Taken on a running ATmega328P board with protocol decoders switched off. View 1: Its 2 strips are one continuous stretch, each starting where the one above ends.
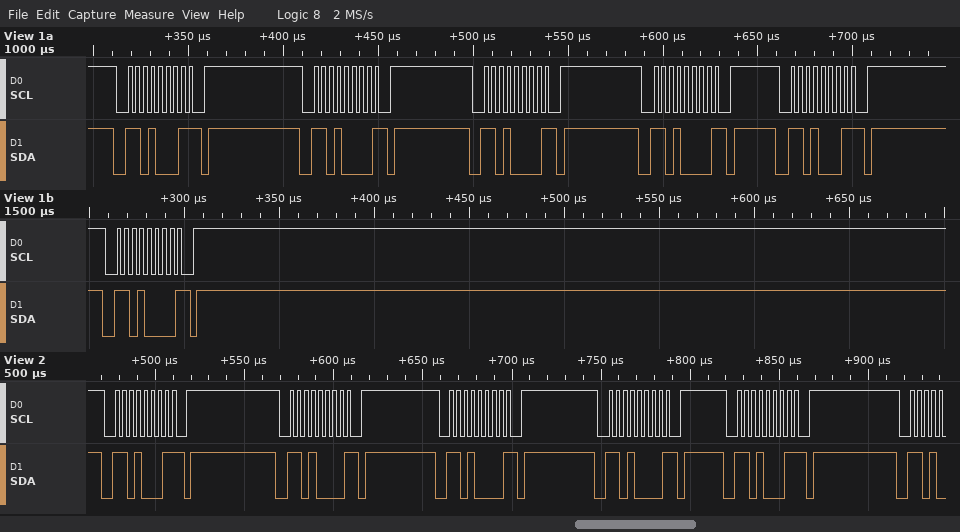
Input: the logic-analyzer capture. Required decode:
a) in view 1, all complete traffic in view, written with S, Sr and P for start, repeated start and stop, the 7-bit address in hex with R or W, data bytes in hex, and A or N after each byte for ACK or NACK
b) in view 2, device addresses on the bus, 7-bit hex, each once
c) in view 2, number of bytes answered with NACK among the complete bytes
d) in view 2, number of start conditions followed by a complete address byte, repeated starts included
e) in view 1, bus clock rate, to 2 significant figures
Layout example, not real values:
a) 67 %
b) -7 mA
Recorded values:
a) S 68R N P S 68W N P S 68W N P S 68W N P S 68R N P S 68W N P
b) 0x68
c) 5
d) 5
e) 250 kHz
